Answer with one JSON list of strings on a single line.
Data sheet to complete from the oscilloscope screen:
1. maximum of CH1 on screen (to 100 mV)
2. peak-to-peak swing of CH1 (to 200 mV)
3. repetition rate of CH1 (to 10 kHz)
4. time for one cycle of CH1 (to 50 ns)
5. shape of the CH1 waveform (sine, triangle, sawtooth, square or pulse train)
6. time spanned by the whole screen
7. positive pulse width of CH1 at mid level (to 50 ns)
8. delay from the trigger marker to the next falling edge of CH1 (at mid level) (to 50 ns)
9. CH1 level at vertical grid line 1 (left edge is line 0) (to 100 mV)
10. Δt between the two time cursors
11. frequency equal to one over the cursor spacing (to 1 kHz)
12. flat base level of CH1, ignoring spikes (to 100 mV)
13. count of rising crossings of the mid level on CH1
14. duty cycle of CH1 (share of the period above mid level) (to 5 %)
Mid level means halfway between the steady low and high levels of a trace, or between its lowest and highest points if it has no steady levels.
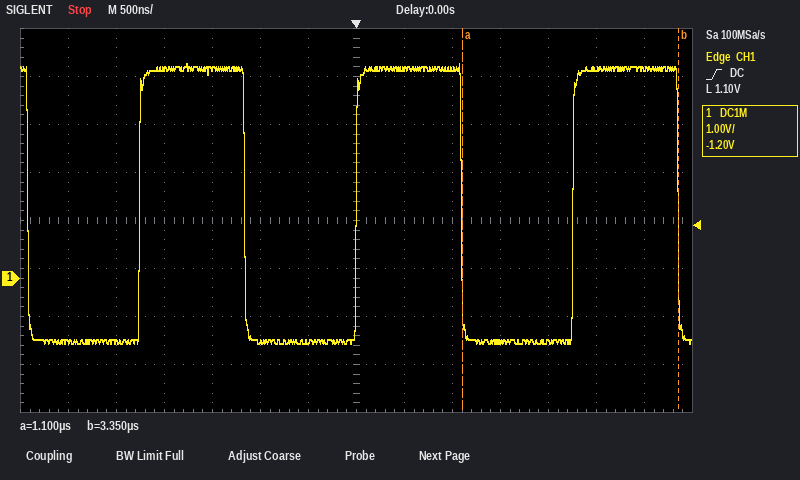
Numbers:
["4.5 V", "5.8 V", "440 kHz", "2.25 µs", "square", "7 µs", "1.10 µs", "1.10 µs", "-1.3 V", "2.25 µs", "444 kHz", "-1.3 V", "3", "50 %"]
